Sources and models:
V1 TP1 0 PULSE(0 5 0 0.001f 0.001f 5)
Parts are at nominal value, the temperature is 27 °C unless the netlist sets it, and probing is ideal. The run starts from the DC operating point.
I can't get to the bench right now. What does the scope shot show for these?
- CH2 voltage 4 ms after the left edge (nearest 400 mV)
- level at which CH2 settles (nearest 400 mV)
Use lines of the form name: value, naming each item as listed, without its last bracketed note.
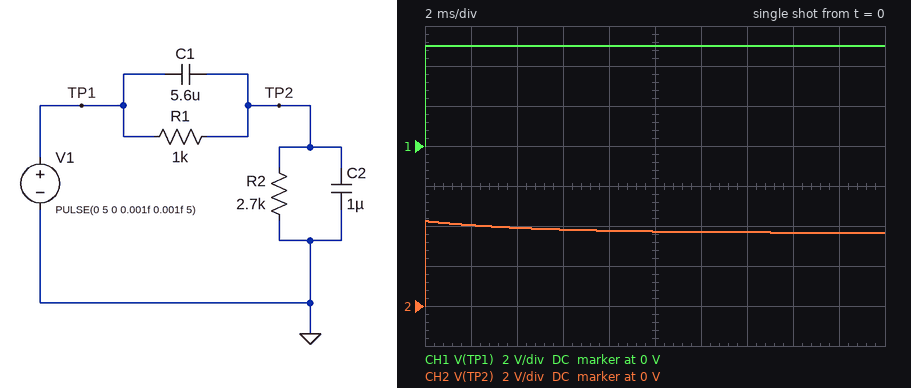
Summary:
CH2 voltage 4 ms after the left edge: 4.0 V
level at which CH2 settles: 3.6 V
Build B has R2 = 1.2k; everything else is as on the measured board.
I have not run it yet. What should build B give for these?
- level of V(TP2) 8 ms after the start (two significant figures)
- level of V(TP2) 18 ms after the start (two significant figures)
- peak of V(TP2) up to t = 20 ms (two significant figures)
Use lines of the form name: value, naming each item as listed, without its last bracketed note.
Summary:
level of V(TP2) 8 ms after the start: 2.9 V
level of V(TP2) 18 ms after the start: 2.7 V
peak of V(TP2) up to t = 20 ms: 4.2 V
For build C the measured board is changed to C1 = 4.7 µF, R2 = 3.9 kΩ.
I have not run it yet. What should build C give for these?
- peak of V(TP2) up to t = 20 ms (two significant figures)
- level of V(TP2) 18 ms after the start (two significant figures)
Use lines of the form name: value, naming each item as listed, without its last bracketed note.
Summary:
peak of V(TP2) up to t = 20 ms: 4.1 V
level of V(TP2) 18 ms after the start: 4.0 V
